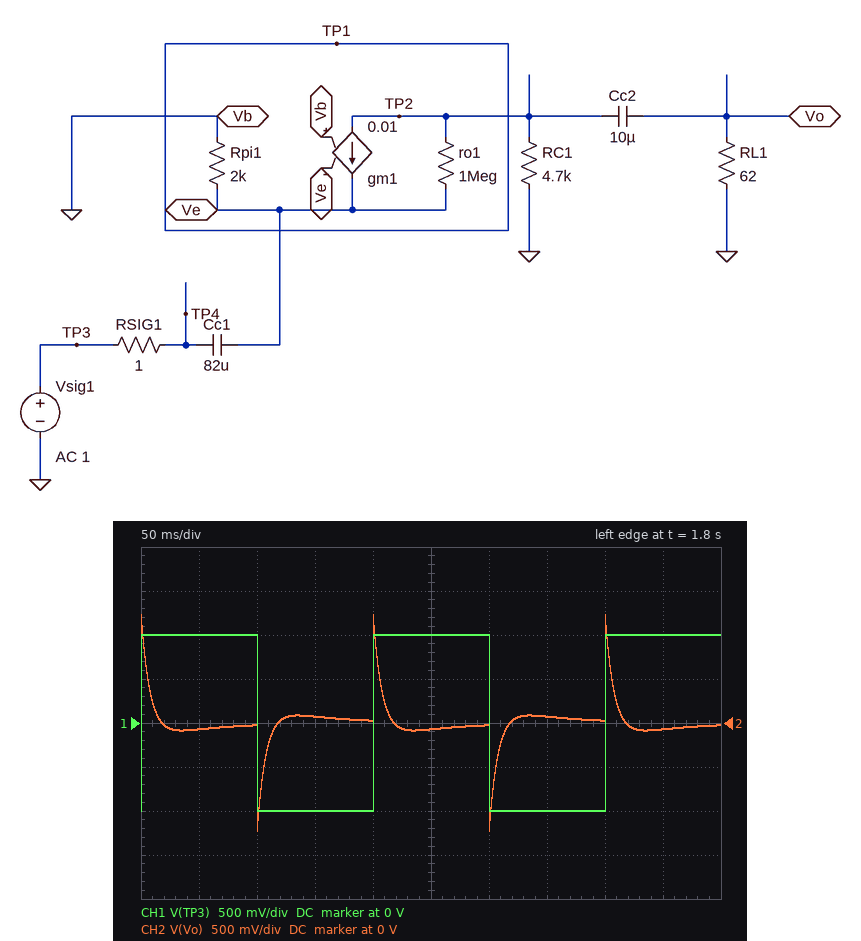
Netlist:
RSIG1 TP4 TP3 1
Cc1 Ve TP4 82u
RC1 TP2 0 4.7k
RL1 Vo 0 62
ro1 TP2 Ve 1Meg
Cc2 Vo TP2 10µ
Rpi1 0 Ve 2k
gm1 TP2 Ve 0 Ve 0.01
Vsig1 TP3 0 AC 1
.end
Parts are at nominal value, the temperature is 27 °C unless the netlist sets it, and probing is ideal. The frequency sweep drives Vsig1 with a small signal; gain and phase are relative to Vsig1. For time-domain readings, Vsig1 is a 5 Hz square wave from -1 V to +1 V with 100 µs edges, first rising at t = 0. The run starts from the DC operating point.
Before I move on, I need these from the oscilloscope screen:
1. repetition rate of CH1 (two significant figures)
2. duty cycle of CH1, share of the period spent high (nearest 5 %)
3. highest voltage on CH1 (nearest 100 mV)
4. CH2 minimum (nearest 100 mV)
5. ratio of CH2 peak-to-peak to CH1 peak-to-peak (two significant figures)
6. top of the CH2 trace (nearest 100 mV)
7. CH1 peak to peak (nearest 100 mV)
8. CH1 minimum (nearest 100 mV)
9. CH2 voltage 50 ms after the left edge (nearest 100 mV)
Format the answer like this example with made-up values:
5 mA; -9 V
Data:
5.0 Hz; 50 %; 1.0 V; -1.2 V; 1.2; 1.2 V; 2.0 V; -1.0 V; -100 mV
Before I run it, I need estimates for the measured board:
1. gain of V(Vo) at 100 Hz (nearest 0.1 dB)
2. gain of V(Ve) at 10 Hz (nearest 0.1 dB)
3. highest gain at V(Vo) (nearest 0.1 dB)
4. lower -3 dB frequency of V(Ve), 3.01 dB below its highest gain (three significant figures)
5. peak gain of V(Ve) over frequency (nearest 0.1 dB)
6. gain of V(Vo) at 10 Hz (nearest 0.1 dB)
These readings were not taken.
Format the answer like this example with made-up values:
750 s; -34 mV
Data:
-4.5 dB; -7.1 dB; -4.4 dB; 20.2 Hz; -0.1 dB; -11.9 dB
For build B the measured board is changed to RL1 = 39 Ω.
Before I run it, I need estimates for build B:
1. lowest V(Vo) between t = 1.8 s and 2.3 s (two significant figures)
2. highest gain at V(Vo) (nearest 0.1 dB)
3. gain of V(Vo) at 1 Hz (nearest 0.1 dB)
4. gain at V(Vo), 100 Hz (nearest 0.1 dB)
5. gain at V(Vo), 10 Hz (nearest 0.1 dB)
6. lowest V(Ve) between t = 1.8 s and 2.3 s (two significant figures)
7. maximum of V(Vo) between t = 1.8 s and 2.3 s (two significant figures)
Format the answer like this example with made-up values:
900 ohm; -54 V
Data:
-780 mV; -8.3 dB; -45.3 dB; -8.5 dB; -15.9 dB; -2.0 V; 780 mV
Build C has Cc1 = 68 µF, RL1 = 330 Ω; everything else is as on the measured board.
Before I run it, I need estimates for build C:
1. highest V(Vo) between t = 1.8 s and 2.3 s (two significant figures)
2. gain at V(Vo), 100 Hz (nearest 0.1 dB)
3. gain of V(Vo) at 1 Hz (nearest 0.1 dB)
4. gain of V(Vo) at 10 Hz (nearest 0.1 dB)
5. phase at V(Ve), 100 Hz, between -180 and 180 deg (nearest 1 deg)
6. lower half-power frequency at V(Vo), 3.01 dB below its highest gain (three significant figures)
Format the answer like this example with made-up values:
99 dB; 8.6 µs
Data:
6.2 V; 9.4 dB; -28.5 dB; 0.9 dB; 14 deg; 24.7 Hz
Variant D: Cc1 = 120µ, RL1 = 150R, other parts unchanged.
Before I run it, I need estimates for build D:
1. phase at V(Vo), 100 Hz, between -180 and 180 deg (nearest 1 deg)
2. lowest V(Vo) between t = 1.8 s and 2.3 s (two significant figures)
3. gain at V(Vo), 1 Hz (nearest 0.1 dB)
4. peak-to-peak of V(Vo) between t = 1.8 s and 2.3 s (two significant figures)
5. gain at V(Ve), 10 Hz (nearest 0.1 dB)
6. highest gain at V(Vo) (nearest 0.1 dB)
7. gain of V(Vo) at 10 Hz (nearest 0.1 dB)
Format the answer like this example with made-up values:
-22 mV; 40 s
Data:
10 deg; -3.0 V; -30.4 dB; 5.9 V; -4.7 dB; 3.2 dB; -1.9 dB
